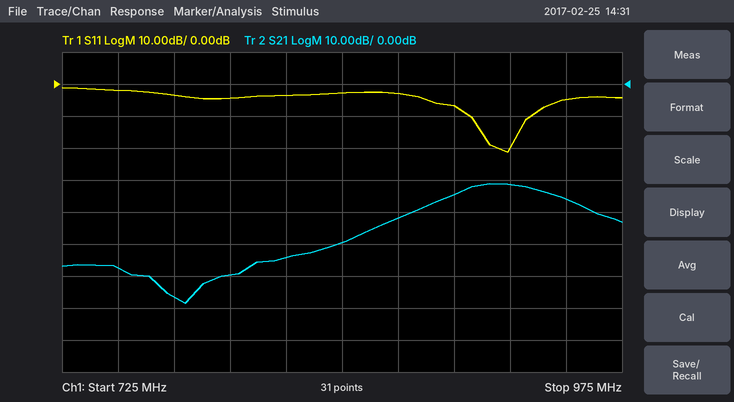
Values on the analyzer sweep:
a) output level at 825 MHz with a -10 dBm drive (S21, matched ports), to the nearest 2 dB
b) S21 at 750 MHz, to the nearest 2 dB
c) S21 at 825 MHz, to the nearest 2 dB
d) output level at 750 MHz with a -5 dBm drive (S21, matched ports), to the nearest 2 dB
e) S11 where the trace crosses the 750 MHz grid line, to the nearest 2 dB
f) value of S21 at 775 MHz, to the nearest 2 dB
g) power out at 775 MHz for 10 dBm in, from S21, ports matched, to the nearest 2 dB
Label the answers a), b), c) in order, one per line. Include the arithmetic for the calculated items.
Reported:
a) -10 dBm + (-54 dB) = -64 dBm
b) -58 dB
c) -54 dB
d) -5 dBm + (-58 dB) = -62 dBm
e) -2 dB
f) -66 dB
g) 10 dBm + (-66 dB) = -56 dBm
